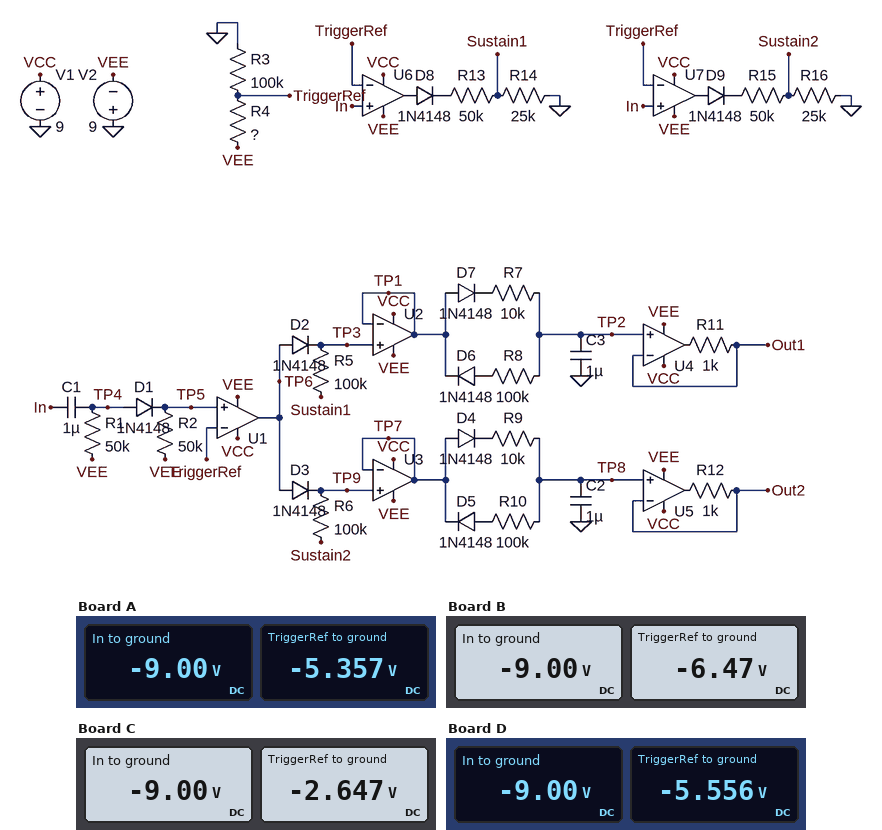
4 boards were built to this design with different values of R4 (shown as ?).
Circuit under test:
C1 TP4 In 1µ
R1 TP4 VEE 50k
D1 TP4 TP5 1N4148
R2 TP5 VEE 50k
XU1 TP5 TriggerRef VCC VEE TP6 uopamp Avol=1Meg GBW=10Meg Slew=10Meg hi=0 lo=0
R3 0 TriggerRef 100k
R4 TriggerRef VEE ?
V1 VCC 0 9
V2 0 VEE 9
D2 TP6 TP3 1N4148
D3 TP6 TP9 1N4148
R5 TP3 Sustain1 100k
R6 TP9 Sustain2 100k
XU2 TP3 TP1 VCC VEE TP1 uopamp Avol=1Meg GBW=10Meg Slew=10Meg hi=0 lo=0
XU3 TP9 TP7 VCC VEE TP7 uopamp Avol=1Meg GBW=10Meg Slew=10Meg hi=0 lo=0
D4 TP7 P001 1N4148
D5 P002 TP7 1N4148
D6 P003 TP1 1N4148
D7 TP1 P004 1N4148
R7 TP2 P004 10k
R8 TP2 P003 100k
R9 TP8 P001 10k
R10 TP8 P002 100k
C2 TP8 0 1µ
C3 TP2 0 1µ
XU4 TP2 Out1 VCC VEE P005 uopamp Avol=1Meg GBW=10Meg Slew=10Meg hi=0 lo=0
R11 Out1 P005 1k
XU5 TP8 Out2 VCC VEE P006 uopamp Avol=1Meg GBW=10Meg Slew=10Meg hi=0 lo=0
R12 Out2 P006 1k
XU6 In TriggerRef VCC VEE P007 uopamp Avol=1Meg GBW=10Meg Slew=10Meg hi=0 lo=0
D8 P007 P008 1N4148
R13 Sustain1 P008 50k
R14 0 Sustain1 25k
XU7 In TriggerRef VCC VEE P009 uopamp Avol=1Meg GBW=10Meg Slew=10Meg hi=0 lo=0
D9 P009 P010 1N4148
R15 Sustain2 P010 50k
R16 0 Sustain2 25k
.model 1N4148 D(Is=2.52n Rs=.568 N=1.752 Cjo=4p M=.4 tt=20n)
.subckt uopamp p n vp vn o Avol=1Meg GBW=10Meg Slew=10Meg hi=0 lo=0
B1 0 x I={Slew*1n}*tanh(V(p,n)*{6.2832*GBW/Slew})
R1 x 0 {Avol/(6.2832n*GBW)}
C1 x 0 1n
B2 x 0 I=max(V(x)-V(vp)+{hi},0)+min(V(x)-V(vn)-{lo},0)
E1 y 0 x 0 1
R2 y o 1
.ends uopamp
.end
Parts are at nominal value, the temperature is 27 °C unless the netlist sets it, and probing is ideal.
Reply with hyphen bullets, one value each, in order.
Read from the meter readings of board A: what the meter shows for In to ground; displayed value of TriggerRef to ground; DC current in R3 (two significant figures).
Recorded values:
- -9.00 V
- -5.357 V
- 54 µA
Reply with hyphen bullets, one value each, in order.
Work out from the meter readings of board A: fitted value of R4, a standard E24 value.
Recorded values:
- 68 kΩ
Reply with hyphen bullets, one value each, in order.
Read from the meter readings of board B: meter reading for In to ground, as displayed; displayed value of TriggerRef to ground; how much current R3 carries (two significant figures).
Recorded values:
- -9.00 V
- -6.47 V
- 65 µA
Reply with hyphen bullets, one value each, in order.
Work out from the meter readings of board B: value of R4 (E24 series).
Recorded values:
- 39 kΩ
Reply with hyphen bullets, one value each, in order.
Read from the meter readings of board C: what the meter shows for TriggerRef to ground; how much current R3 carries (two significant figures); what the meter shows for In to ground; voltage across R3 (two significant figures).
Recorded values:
- -2.647 V
- 26 µA
- -9.00 V
- 2.6 V
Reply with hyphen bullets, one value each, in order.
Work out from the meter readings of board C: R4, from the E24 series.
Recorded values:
- 240 kΩ
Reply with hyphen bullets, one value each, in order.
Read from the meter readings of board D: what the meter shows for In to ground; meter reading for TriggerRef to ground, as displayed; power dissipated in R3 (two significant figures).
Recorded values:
- -9.00 V
- -5.556 V
- 310 µW
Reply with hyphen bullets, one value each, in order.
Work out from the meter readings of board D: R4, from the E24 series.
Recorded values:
- 62 kΩ
